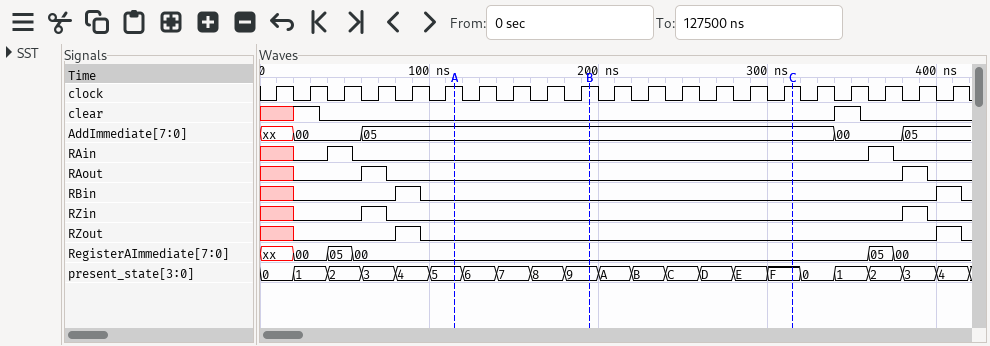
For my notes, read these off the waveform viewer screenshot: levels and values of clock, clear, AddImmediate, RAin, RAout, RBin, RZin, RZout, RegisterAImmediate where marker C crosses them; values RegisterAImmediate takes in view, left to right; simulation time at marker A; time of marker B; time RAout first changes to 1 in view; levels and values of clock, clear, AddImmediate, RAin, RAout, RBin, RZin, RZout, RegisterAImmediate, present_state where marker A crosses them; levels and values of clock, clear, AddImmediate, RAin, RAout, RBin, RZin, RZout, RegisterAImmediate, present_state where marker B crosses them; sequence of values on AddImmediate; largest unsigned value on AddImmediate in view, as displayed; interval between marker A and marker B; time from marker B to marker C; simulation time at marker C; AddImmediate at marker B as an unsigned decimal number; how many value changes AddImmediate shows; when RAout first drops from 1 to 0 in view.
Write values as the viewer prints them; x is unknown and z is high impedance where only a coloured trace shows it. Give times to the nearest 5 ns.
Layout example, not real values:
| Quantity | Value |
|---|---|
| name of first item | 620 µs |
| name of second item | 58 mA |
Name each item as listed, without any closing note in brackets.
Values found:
| Quantity | Value |
|---|---|
| levels and values of clock, clear, AddImmediate, RAin, RAout, RBin, RZin, RZout, RegisterAImmediate where marker C crosses them | clock=1, clear=0, AddImmediate=05, RAin=0, RAout=0, RBin=0, RZin=0, RZout=0, RegisterAImmediate=00 |
| values RegisterAImmediate takes in view, left to right | xx, 00, 05, 00, 05, 00 |
| simulation time at marker A | 115 ns |
| time of marker B | 195 ns |
| time RAout first changes to 1 in view | 60 ns |
| levels and values of clock, clear, AddImmediate, RAin, RAout, RBin, RZin, RZout, RegisterAImmediate, present_state where marker A crosses them | clock=1, clear=0, AddImmediate=05, RAin=0, RAout=0, RBin=0, RZin=0, RZout=0, RegisterAImmediate=00, present_state=5 |
| levels and values of clock, clear, AddImmediate, RAin, RAout, RBin, RZin, RZout, RegisterAImmediate, present_state where marker B crosses them | clock=1, clear=0, AddImmediate=05, RAin=0, RAout=0, RBin=0, RZin=0, RZout=0, RegisterAImmediate=00, present_state=9 |
| sequence of values on AddImmediate | xx, 00, 05, 00, 05 |
| largest unsigned value on AddImmediate in view, as displayed | 05 |
| interval between marker A and marker B | 80 ns |
| time from marker B to marker C | 120 ns |
| simulation time at marker C | 315 ns |
| AddImmediate at marker B as an unsigned decimal number | 5 |
| how many value changes AddImmediate shows | 4 |
| when RAout first drops from 1 to 0 in view | 75 ns |
